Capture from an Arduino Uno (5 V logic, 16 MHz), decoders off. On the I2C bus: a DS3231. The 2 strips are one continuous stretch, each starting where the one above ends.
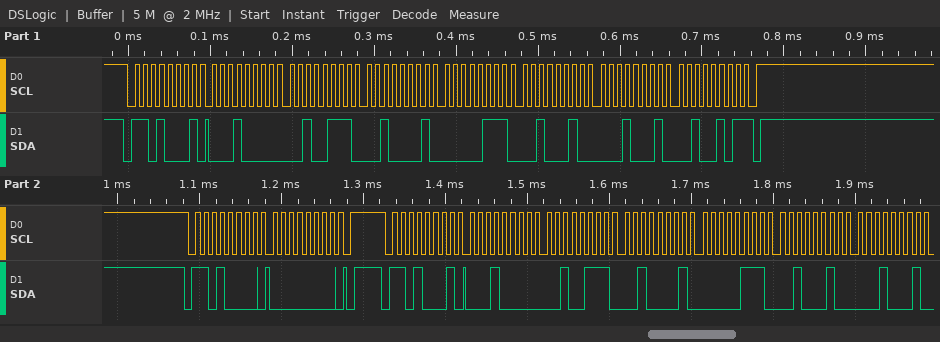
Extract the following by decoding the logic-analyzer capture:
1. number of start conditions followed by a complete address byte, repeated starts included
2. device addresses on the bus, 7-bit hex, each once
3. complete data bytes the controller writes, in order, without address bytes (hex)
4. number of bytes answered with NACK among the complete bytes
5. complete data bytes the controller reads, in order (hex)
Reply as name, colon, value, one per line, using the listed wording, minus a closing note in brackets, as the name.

number of start conditions followed by a complete address byte, repeated starts included: 3
device addresses on the bus, 7-bit hex, each once: 0x68
complete data bytes the controller writes, in order, without address bytes: 00
number of bytes answered with NACK among the complete bytes: 1
complete data bytes the controller reads, in order: 10 27 21 07 22 11 25 10 27 21 07 22 11
